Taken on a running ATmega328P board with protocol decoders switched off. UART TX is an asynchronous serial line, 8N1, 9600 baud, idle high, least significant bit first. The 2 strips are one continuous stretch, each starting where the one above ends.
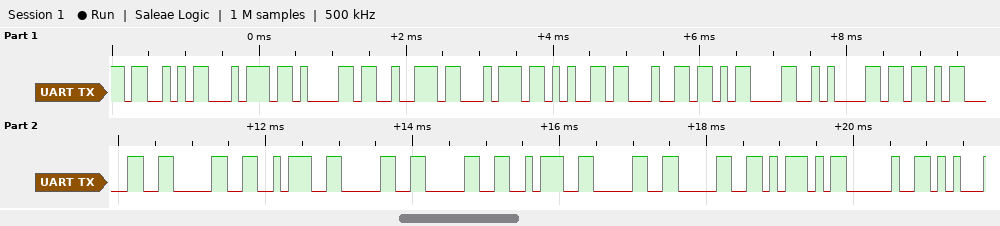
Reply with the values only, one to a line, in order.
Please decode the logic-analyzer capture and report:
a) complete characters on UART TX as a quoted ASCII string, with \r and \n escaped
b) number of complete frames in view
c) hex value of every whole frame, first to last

"Started\r\n[00:00:00] "
20
53 74 61 72 74 65 64 0D 0A 5B 30 30 3A 30 30 3A 30 30 5D 20
